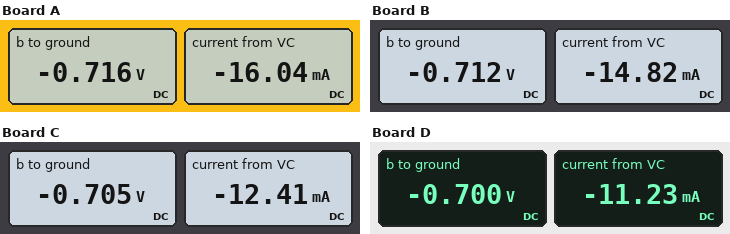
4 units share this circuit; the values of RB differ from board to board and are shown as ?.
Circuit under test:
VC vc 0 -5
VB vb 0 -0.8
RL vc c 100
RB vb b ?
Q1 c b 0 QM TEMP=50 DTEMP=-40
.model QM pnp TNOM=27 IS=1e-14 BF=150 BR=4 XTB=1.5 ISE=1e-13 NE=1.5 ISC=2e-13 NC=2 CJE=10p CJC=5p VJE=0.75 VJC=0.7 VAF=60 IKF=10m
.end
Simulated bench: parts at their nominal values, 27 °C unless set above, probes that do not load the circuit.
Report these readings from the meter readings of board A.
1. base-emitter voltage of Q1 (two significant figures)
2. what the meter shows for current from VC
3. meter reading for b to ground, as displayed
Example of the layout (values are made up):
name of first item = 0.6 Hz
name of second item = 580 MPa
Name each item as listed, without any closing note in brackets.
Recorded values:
base-emitter voltage of Q1 = -720 mV
what the meter shows for current from VC = -16.04 mA
meter reading for b to ground, as displayed = -0.716 V
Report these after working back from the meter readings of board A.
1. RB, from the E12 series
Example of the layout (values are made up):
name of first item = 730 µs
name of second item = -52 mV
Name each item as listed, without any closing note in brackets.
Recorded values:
RB, from the E12 series = 330 Ω
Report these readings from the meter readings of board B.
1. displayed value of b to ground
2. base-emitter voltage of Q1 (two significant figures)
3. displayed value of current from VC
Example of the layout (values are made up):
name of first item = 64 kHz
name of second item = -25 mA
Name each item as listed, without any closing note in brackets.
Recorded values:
displayed value of b to ground = -0.712 V
base-emitter voltage of Q1 = -710 mV
displayed value of current from VC = -14.82 mA
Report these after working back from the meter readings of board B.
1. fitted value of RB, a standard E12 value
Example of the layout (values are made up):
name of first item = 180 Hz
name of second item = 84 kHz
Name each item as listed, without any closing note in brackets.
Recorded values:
fitted value of RB, a standard E12 value = 390 Ω
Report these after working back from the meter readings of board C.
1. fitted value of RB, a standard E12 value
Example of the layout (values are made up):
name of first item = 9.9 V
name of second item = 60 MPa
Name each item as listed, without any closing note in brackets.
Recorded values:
fitted value of RB, a standard E12 value = 560 Ω
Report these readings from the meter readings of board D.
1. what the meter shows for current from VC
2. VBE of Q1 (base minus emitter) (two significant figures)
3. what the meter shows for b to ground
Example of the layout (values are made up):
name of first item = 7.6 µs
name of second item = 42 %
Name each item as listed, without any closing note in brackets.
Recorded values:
what the meter shows for current from VC = -11.23 mA
VBE of Q1 (base minus emitter) = -700 mV
what the meter shows for b to ground = -0.700 V
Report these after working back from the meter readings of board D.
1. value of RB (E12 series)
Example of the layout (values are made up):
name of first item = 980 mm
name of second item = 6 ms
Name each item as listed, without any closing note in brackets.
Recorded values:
value of RB = 680 Ω
